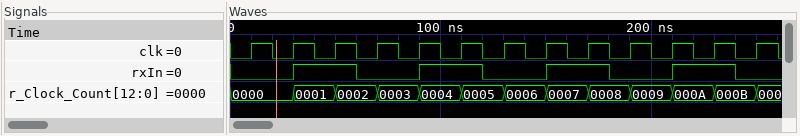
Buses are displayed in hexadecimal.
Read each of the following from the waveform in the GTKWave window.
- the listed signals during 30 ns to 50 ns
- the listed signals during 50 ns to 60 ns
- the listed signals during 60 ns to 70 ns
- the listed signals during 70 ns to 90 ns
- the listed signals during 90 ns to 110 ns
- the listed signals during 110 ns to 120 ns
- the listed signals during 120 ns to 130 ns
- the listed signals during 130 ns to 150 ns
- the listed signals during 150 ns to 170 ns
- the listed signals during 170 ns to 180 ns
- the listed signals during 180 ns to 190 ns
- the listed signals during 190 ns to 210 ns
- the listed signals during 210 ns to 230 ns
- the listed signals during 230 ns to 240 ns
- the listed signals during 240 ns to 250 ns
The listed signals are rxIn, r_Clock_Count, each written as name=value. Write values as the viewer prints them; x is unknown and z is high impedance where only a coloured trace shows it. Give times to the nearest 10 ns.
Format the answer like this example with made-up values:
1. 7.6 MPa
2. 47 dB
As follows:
1. rxIn=1, r_Clock_Count=0001
2. rxIn=1, r_Clock_Count=0002
3. rxIn=0, r_Clock_Count=0002
4. rxIn=0, r_Clock_Count=0003
5. rxIn=1, r_Clock_Count=0004
6. rxIn=1, r_Clock_Count=0005
7. rxIn=0, r_Clock_Count=0005
8. rxIn=0, r_Clock_Count=0006
9. rxIn=1, r_Clock_Count=0007
10. rxIn=1, r_Clock_Count=0008
11. rxIn=0, r_Clock_Count=0008
12. rxIn=0, r_Clock_Count=0009
13. rxIn=1, r_Clock_Count=000A
14. rxIn=1, r_Clock_Count=000B
15. rxIn=0, r_Clock_Count=000B
